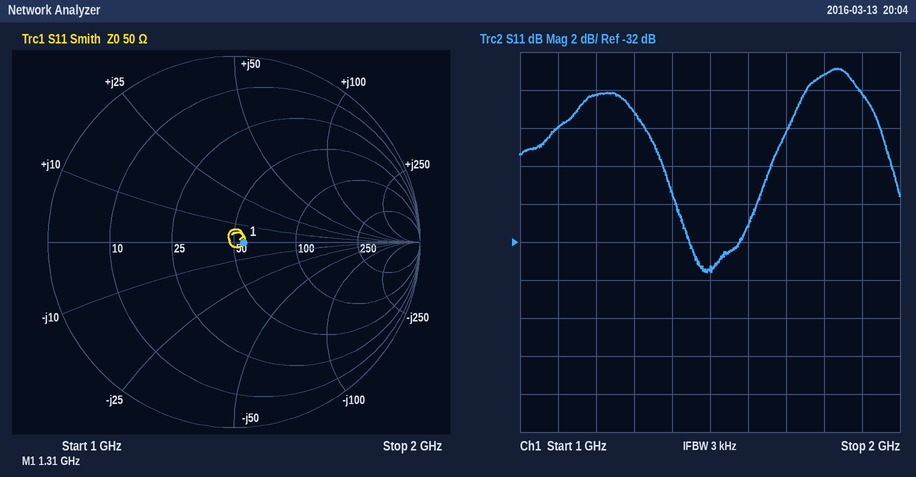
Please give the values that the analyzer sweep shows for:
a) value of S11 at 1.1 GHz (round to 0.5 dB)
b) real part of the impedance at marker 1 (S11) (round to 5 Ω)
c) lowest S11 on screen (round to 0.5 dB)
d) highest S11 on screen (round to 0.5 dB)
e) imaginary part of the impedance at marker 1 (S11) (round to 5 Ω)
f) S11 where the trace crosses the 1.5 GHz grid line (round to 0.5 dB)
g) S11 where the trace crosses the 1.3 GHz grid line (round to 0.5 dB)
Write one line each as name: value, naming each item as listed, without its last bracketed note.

value of S11 at 1.1 GHz: -26.0 dB
real part of the impedance at marker 1 (S11): 55 Ω
lowest S11 on screen: -33.5 dB
highest S11 on screen: -23.0 dB
imaginary part of the impedance at marker 1 (S11): 0 Ω
S11 where the trace crosses the 1.5 GHz grid line: -33.5 dB
S11 where the trace crosses the 1.3 GHz grid line: -25.0 dB
